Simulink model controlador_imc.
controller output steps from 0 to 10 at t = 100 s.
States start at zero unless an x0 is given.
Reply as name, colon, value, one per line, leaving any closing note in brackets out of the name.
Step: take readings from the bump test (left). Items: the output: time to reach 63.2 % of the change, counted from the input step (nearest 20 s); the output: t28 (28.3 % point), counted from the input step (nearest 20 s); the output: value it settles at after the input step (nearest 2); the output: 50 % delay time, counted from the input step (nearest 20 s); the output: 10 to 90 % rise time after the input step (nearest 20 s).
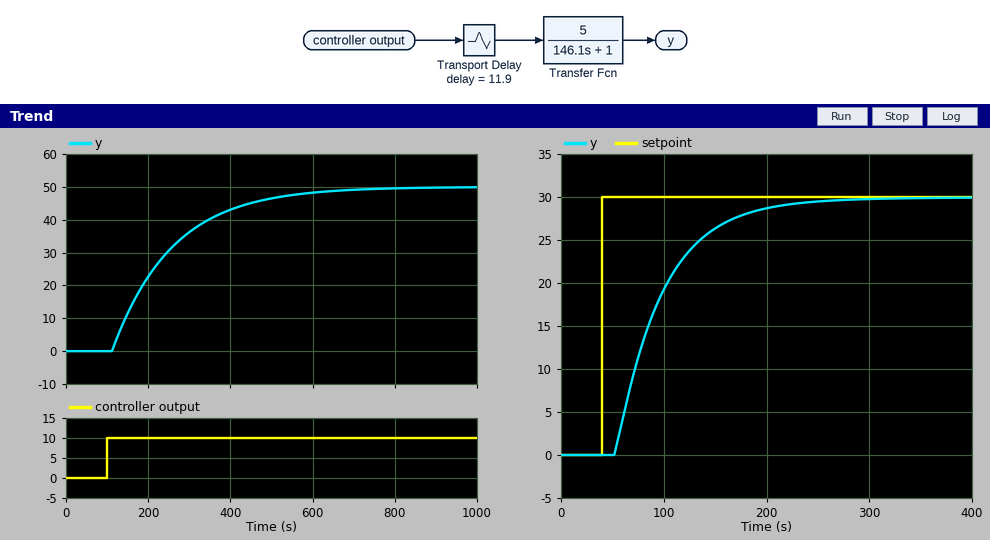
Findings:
the output: time to reach 63.2 % of the change, counted from the input step: 160 s
the output: t28 (28.3 % point), counted from the input step: 60 s
the output: value it settles at after the input step: 50
the output: 50 % delay time, counted from the input step: 120 s
the output: 10 to 90 % rise time after the input step: 320 s
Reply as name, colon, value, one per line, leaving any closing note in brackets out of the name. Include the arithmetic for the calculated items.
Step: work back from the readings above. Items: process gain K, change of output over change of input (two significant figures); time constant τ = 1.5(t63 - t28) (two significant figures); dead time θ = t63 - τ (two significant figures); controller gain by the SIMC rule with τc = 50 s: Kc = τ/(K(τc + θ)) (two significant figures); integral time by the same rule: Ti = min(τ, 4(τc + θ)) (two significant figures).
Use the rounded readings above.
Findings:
process gain K, change of output over change of input: (50 - 0) / 10 = 5.0
time constant τ = 1.5(t63 - t28): 1.5 × (160 - 60) = 150 s
dead time θ = t63 - τ: 160 - 150 = 10 s
controller gain by the SIMC rule with τc = 50 s: Kc = τ/(K(τc + θ)): 150 / (5 × (50 + 10)) = 0.50
integral time by the same rule: Ti = min(τ, 4(τc + θ)): min(150, 4 × (50 + 10)) = 150 s
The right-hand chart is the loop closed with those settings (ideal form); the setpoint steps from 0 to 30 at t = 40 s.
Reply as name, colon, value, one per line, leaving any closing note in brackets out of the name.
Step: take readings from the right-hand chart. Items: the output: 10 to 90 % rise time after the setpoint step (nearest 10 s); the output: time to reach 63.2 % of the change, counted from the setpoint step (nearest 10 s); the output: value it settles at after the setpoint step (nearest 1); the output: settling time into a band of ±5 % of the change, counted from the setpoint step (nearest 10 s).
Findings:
the output: 10 to 90 % rise time after the setpoint step: 100 s
the output: time to reach 63.2 % of the change, counted from the setpoint step: 60 s
the output: value it settles at after the setpoint step: 30
the output: settling time into a band of ±5 % of the change, counted from the setpoint step: 150 s
